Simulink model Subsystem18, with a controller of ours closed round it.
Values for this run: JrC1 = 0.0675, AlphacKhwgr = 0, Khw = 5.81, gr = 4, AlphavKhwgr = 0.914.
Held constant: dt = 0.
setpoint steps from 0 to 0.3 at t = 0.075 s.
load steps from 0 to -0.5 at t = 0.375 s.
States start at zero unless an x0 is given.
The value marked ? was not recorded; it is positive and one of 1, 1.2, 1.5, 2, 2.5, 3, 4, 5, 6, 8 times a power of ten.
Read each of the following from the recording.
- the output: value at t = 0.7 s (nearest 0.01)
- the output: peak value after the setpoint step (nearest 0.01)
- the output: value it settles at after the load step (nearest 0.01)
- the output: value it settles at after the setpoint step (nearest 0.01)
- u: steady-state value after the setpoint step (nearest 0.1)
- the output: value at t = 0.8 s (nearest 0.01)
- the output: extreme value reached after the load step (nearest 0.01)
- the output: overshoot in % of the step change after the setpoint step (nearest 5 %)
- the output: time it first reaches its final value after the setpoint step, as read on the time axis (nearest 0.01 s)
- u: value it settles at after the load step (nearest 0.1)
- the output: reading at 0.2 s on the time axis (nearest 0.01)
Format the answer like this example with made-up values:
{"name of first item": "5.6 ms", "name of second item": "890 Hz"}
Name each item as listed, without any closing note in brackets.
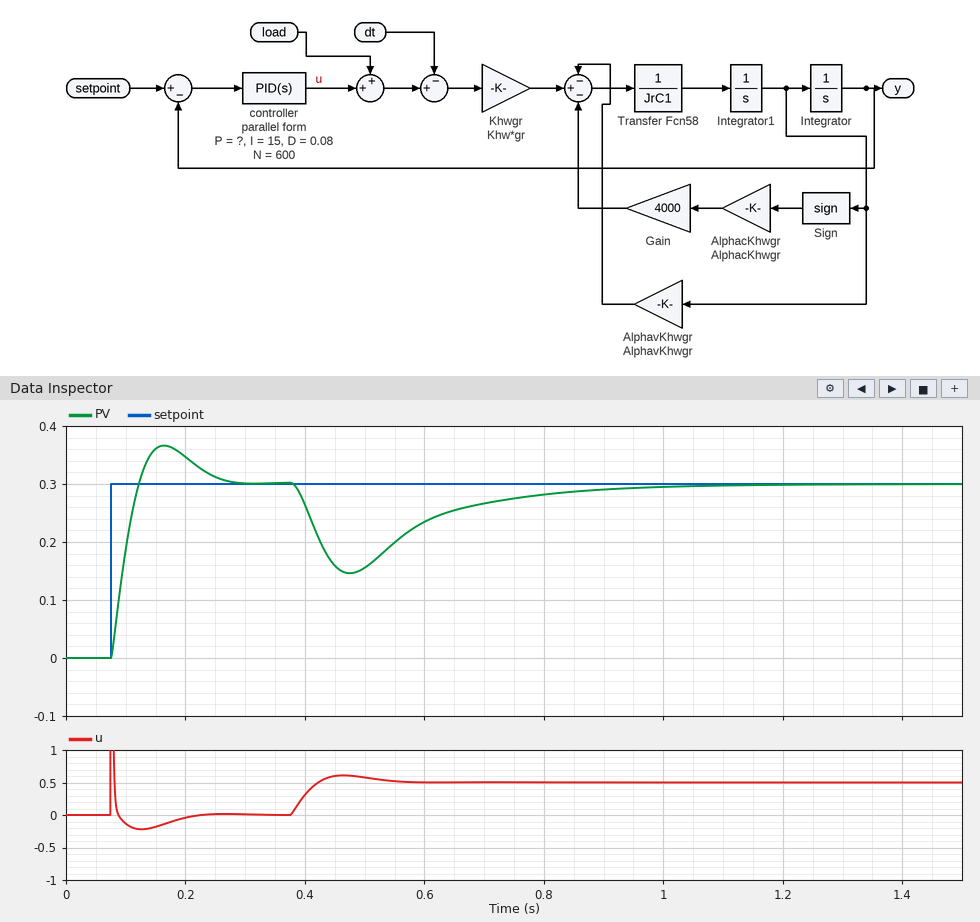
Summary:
{"the output: value at t = 0.7 s": "0.27", "the output: peak value after the setpoint step": "0.37", "the output: value it settles at after the load step": "0.30", "the output: value it settles at after the setpoint step": "0.30", "u: steady-state value after the setpoint step": "0.0", "the output: value at t = 0.8 s": "0.28", "the output: extreme value reached after the load step": "0.15", "the output: overshoot in % of the step change after the setpoint step": "20 %", "the output: time it first reaches its final value after the setpoint step, as read on the time axis": "0.12 s", "u: value it settles at after the load step": "0.5", "the output: reading at 0.2 s on the time axis": "0.35"}
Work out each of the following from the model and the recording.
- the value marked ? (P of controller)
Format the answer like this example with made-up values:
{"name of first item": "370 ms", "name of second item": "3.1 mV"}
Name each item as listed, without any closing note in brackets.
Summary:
{"the value marked ?": "3"}
